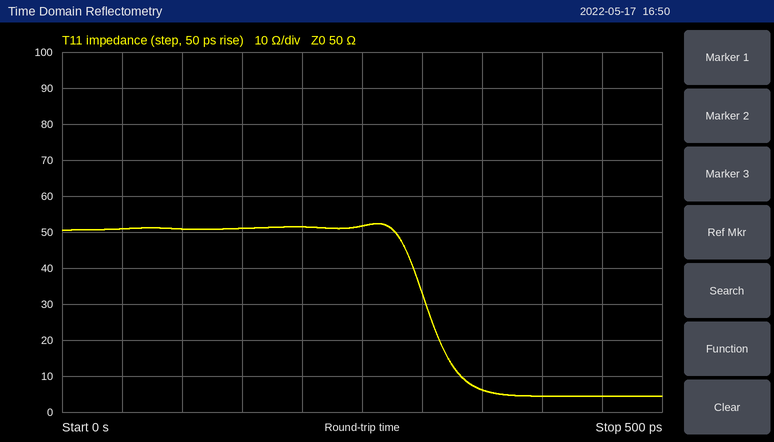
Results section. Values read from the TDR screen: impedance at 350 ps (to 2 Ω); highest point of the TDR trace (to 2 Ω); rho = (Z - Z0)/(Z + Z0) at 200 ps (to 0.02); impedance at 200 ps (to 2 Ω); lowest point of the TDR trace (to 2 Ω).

6 Ω
52 Ω
+0.02
52 Ω
4 Ω
